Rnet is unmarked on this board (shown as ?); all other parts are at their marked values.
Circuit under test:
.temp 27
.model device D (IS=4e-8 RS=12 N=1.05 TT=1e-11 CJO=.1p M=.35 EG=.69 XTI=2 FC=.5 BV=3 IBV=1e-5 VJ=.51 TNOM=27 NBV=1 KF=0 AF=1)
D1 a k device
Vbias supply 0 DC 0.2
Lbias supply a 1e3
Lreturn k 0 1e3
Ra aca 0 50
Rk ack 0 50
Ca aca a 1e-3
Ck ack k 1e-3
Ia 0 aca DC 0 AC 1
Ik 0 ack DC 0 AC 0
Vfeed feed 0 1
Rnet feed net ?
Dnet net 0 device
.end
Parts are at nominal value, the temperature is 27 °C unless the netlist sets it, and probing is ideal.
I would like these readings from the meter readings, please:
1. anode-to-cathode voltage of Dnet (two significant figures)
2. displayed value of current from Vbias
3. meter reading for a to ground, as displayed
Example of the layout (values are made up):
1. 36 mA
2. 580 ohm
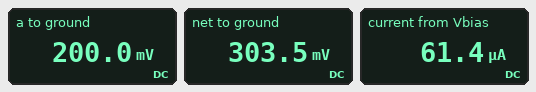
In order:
1. 300 mV
2. 61.4 µA
3. 200.0 mV
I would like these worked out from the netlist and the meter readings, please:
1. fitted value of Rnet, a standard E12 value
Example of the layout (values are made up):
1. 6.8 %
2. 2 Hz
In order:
1. 470 Ω
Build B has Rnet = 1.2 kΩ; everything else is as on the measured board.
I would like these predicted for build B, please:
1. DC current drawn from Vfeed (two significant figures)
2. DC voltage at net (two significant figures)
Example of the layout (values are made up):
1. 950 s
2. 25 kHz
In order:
1. 610 µA
2. 270 mV
